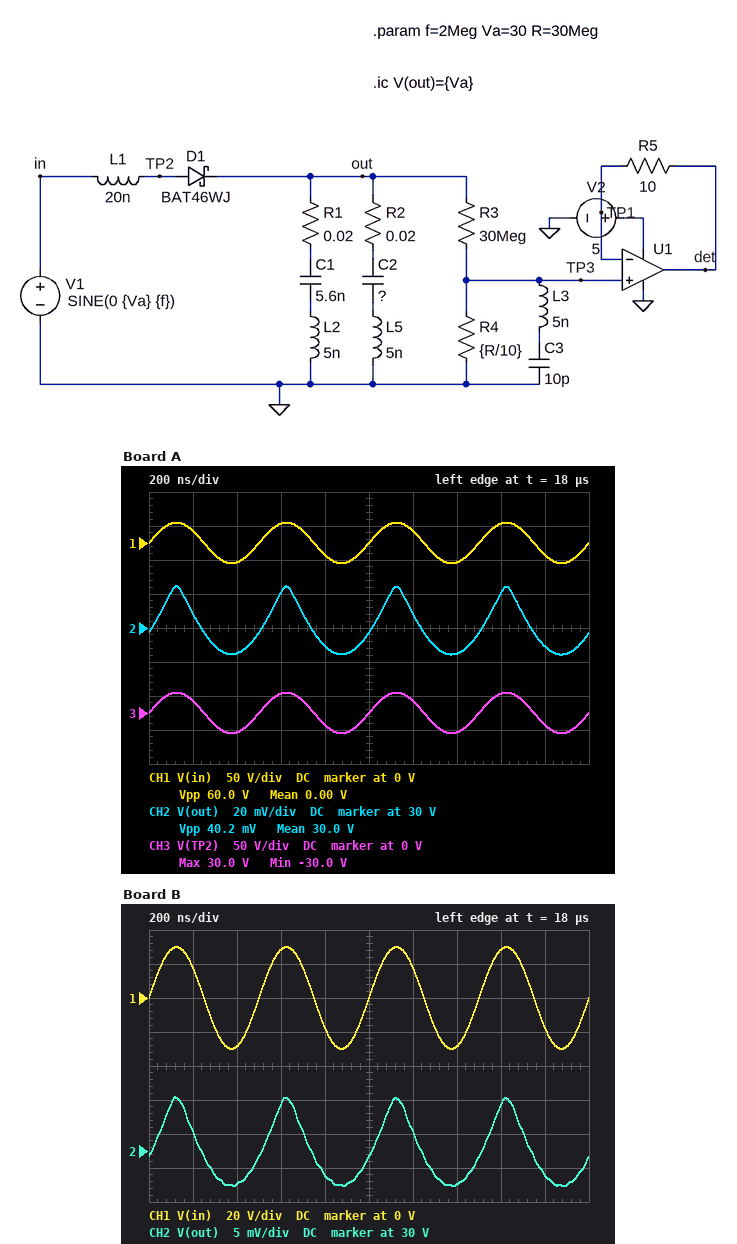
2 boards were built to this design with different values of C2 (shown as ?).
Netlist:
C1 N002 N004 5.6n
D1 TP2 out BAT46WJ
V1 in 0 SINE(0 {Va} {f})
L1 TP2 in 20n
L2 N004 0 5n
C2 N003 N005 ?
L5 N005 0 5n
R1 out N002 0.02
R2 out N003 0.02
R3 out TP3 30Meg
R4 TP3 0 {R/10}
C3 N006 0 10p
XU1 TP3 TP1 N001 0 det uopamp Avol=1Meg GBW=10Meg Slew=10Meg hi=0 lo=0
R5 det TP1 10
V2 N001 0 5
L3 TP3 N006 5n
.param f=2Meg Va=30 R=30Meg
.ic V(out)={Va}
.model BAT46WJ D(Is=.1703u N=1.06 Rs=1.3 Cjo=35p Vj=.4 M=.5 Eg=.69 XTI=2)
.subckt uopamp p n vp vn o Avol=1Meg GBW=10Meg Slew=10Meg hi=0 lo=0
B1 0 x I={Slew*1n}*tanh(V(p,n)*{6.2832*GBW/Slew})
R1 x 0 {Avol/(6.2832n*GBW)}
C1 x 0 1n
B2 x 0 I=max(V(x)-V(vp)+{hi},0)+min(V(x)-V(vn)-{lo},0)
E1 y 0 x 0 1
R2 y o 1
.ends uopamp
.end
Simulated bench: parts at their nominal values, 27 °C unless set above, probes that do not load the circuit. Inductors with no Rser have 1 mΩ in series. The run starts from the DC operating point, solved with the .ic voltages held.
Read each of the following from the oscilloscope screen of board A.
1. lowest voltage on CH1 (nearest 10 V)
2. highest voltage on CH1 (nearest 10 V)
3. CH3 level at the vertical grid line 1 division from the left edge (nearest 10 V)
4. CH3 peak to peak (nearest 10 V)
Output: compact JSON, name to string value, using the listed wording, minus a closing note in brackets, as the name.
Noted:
{"lowest voltage on CH1": "-30 V", "highest voltage on CH1": "30 V", "CH3 level at the vertical grid line 1 division from the left edge": "20 V", "CH3 peak to peak": "60 V"}
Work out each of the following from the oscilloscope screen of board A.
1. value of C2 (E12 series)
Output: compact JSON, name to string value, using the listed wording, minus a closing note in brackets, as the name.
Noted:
{"value of C2": "2.2 nF"}
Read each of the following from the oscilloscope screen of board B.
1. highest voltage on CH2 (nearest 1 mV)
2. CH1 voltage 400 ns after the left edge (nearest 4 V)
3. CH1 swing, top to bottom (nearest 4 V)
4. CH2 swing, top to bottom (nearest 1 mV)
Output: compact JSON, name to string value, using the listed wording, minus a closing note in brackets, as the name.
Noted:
{"highest voltage on CH2": "30.008 V", "CH1 voltage 400 ns after the left edge": "-28 V", "CH1 swing, top to bottom": "60 V", "CH2 swing, top to bottom": "13 mV"}
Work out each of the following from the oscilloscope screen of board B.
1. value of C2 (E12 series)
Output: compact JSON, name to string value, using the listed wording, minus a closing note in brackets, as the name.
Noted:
{"value of C2": "18 nF"}
